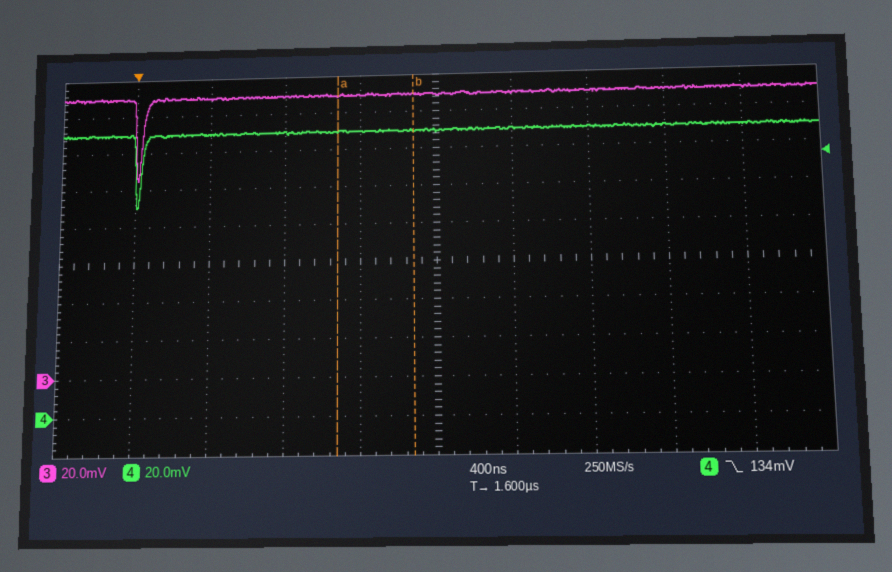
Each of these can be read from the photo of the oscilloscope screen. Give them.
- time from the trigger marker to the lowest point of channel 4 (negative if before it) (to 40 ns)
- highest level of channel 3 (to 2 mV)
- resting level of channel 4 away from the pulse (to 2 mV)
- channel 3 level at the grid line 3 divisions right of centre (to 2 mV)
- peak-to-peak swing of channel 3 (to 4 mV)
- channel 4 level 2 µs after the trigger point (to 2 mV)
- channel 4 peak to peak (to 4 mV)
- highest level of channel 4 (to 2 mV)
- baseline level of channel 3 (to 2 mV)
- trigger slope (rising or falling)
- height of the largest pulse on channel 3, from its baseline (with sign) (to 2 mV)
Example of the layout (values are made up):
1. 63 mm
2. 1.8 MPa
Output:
1. 0 ns
2. 150 mV
3. 150 mV
4. 150 mV
5. 44 mV
6. 150 mV
7. 40 mV
8. 150 mV
9. 150 mV
10. falling
11. -44 mV
